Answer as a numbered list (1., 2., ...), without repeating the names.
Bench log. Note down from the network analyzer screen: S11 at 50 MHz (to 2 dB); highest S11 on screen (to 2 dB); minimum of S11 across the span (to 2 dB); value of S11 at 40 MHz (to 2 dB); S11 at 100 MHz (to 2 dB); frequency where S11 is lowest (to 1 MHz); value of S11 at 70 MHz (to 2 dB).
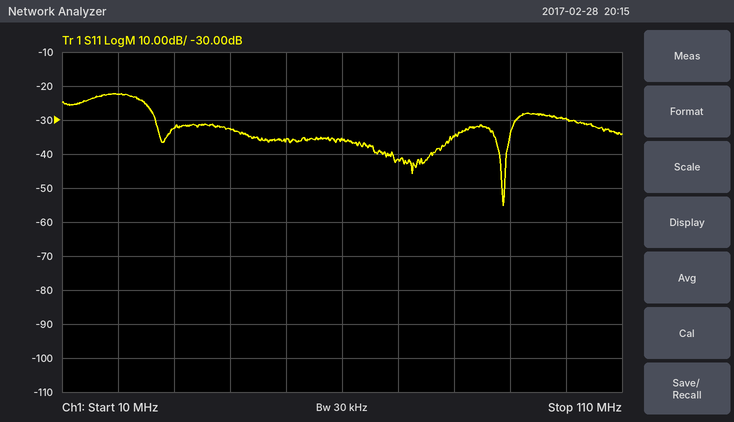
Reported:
1. -36 dB
2. -22 dB
3. -56 dB
4. -32 dB
5. -30 dB
6. 89 MHz
7. -42 dB
